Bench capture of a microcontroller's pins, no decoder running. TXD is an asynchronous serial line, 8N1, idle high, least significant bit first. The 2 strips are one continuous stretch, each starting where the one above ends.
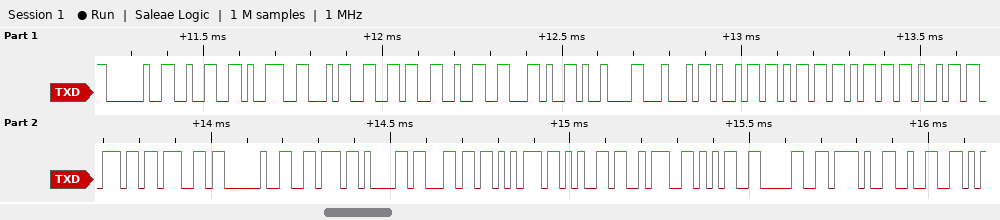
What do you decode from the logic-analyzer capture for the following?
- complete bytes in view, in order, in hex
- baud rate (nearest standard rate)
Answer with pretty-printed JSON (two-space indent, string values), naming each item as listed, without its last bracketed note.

{
  "complete bytes in view, in order, in hex": "20 32 39 34 36 32 2C 09 44 69 6D 6D 69 6E 67 20 76 61 6C 75 65 3A 35 30 2F 32",
  "baud rate": "57600 baud"
}
